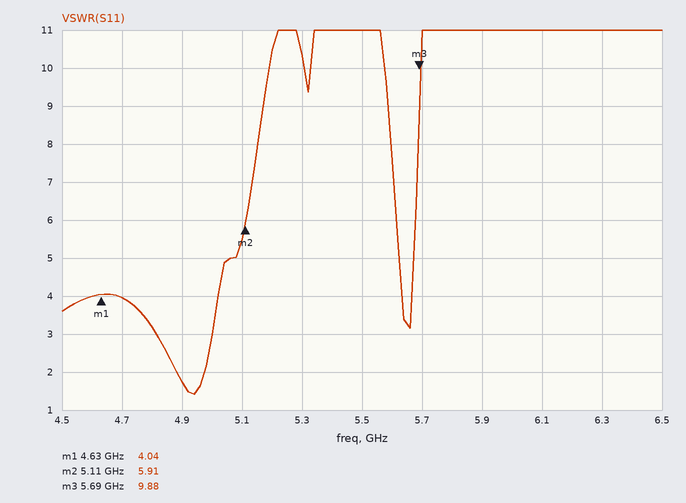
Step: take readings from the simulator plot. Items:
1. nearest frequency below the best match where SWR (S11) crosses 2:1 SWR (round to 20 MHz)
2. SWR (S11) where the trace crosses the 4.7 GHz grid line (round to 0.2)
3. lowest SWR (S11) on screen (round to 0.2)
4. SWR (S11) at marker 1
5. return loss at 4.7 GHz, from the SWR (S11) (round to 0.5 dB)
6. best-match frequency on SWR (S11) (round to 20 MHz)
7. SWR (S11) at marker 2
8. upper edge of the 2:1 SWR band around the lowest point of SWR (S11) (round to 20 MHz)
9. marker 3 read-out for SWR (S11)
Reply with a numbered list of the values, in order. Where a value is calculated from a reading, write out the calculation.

1. 4.88 GHz
2. 4.0
3. 1.4
4. 4.04
5. −20 log10((4 − 1)/(4 + 1)) ≈ 4.44 dB, so 4.5 dB to the nearest 0.5 dB
6. 4.94 GHz
7. 5.91
8. 4.98 GHz
9. 9.88
